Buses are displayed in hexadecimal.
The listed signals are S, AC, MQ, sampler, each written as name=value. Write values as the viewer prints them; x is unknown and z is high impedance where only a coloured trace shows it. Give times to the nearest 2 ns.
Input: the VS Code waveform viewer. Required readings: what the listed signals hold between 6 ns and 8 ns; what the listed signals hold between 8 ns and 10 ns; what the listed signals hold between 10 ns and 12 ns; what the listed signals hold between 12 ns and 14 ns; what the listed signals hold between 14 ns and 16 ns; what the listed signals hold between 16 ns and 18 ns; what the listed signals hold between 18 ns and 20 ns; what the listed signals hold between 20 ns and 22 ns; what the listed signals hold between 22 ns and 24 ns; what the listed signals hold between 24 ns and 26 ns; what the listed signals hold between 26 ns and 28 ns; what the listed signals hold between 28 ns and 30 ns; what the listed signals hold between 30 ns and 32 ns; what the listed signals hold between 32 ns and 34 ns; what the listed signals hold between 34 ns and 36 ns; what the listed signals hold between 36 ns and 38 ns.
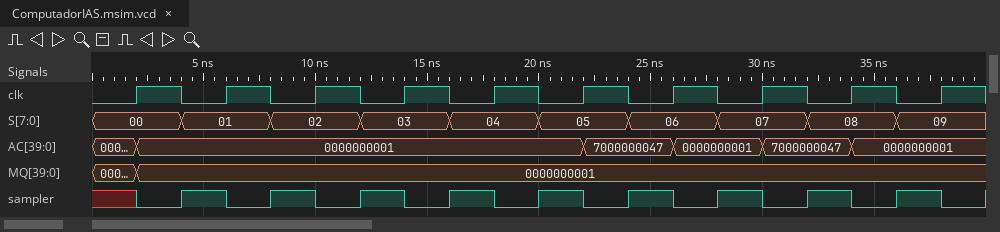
S=01, AC=0000000001, MQ=0000000001, sampler=0
S=02, AC=0000000001, MQ=0000000001, sampler=1
S=02, AC=0000000001, MQ=0000000001, sampler=0
S=03, AC=0000000001, MQ=0000000001, sampler=1
S=03, AC=0000000001, MQ=0000000001, sampler=0
S=04, AC=0000000001, MQ=0000000001, sampler=1
S=04, AC=0000000001, MQ=0000000001, sampler=0
S=05, AC=0000000001, MQ=0000000001, sampler=1
S=05, AC=7000000047, MQ=0000000001, sampler=0
S=06, AC=7000000047, MQ=0000000001, sampler=1
S=06, AC=0000000001, MQ=0000000001, sampler=0
S=07, AC=0000000001, MQ=0000000001, sampler=1
S=07, AC=7000000047, MQ=0000000001, sampler=0
S=08, AC=7000000047, MQ=0000000001, sampler=1
S=08, AC=0000000001, MQ=0000000001, sampler=0
S=09, AC=0000000001, MQ=0000000001, sampler=1
